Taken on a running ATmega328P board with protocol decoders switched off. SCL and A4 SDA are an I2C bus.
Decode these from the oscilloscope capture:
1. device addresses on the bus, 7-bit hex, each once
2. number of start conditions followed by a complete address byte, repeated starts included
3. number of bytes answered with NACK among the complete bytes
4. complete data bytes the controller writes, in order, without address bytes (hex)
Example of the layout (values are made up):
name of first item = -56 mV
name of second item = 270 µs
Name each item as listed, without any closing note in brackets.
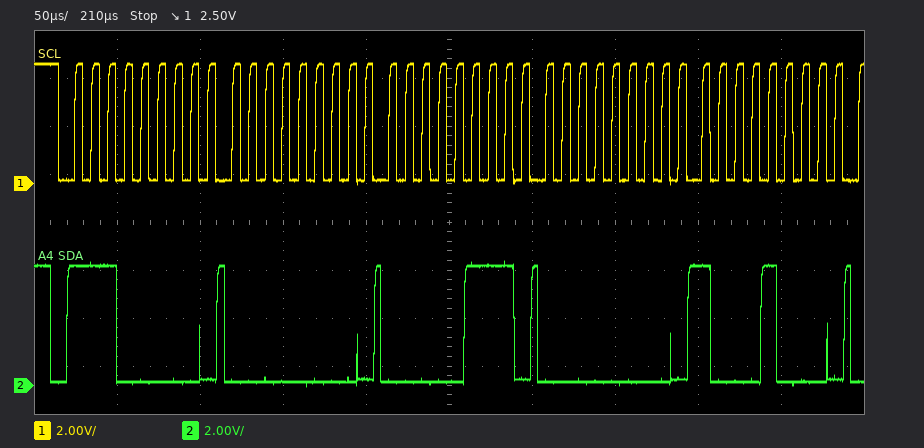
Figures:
device addresses on the bus, 7-bit hex, each once = 0x70
number of start conditions followed by a complete address byte, repeated starts included = 1
number of bytes answered with NACK among the complete bytes = 0
complete data bytes the controller writes, in order, without address bytes = 00 07 00 88
